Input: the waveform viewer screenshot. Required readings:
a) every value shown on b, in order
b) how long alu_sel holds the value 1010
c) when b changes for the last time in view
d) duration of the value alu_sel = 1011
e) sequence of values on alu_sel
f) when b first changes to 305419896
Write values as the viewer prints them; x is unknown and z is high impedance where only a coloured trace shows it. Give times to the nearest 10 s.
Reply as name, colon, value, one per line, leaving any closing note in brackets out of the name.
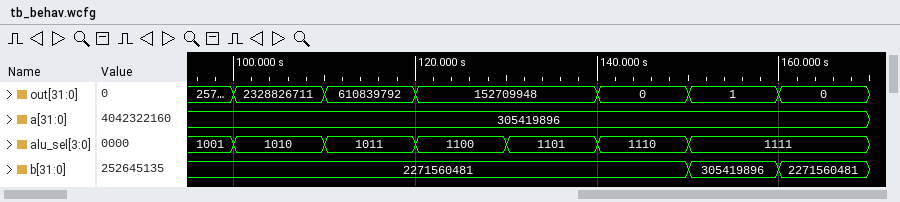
every value shown on b, in order: 2271560481, 305419896, 2271560481
how long alu_sel holds the value 1010: 10 s
when b changes for the last time in view: 160 s
duration of the value alu_sel = 1011: 10 s
sequence of values on alu_sel: 1001, 1010, 1011, 1100, 1101, 1110, 1111
when b first changes to 305419896: 150 s
